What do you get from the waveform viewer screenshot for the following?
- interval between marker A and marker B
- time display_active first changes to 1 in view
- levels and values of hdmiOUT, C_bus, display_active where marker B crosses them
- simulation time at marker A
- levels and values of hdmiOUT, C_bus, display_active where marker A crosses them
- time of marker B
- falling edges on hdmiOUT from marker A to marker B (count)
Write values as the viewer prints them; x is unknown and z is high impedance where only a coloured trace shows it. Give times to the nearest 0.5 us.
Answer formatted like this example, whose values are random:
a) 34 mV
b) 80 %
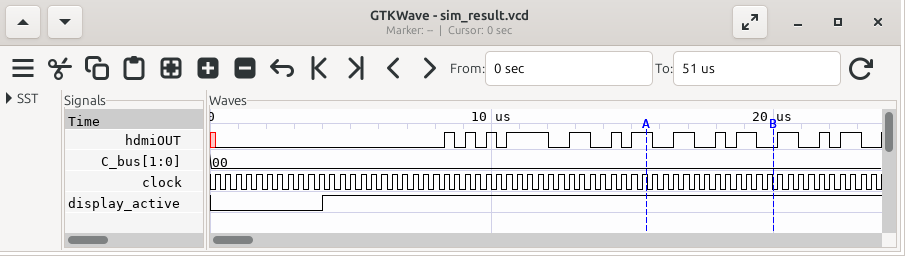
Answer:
a) 4.5 us
b) 4 us
c) hdmiOUT=0, C_bus=00, display_active=1
d) 15.5 us
e) hdmiOUT=1, C_bus=00, display_active=1
f) 20 us
g) 4
